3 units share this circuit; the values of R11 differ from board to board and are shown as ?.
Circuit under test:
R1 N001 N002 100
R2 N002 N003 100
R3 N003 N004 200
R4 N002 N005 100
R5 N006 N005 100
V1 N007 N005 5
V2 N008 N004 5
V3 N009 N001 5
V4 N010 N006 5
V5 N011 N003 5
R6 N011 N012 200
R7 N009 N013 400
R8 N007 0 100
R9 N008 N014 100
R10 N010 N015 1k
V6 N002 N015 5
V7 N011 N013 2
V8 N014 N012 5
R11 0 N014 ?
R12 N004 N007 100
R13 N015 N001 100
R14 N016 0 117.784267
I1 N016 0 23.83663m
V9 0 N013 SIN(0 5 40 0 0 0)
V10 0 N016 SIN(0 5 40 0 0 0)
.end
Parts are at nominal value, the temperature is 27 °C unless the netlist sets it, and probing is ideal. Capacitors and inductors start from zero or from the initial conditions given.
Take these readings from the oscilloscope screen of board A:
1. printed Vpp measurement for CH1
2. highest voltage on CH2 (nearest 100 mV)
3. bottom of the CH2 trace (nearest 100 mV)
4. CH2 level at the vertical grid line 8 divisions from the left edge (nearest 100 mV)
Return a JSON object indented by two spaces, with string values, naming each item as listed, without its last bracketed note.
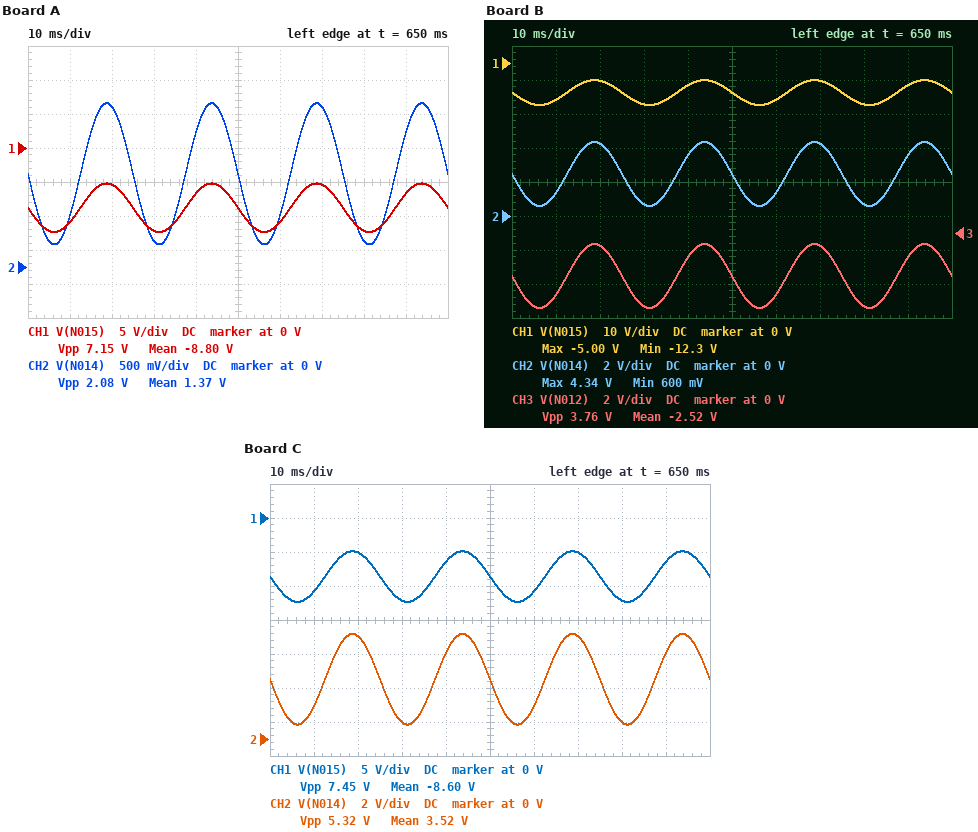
{
  "printed Vpp measurement for CH1": "7.15 V",
  "highest voltage on CH2": "2.4 V",
  "bottom of the CH2 trace": "300 mV",
  "CH2 level at the vertical grid line 8 divisions from the left edge": "400 mV"
}
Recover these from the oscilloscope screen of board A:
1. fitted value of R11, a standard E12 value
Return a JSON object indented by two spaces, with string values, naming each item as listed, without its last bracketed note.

{
  "fitted value of R11, a standard E12 value": "33 Ω"
}
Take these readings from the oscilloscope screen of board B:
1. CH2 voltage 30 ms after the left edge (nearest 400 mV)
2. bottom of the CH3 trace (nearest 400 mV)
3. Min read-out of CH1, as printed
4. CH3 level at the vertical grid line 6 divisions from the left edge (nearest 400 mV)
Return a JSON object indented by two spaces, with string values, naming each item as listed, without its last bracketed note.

{
  "CH2 voltage 30 ms after the left edge": "800 mV",
  "bottom of the CH3 trace": "-4.4 V",
  "Min read-out of CH1, as printed": "-12.3 V",
  "CH3 level at the vertical grid line 6 divisions from the left edge": "-3.6 V"
}
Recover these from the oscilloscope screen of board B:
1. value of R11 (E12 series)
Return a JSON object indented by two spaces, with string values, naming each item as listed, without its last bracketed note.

{
  "value of R11": "82 Ω"
}
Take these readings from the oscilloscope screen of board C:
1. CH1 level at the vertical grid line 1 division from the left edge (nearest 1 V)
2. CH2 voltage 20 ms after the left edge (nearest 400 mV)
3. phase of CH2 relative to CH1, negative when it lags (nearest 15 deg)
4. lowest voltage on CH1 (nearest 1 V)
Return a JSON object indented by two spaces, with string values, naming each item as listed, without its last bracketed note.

{
  "CH1 level at the vertical grid line 1 division from the left edge": "-11 V",
  "CH2 voltage 20 ms after the left edge": "6.0 V",
  "phase of CH2 relative to CH1, negative when it lags": "0 deg",
  "lowest voltage on CH1": "-12 V"
}
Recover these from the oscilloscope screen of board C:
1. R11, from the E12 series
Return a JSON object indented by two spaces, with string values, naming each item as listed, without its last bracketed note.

{
  "R11, from the E12 series": "180 Ω"
}
